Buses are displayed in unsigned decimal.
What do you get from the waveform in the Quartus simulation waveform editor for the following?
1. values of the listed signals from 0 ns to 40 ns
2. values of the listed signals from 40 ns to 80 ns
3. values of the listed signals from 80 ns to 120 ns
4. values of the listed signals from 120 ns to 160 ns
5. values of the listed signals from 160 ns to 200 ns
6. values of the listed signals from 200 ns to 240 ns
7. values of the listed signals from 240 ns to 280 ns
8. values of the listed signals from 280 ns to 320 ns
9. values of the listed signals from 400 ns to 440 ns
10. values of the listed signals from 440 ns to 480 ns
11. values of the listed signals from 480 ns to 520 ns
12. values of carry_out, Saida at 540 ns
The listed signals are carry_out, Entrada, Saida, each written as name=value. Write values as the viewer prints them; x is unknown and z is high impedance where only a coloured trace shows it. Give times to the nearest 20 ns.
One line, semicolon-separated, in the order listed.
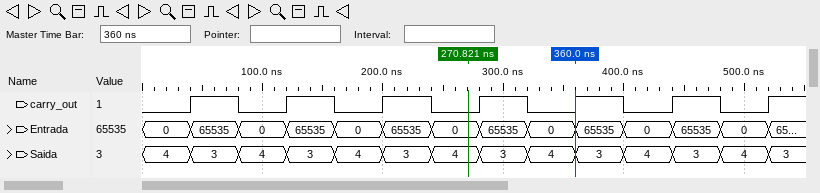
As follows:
carry_out=0, Entrada=0, Saida=4; carry_out=1, Entrada=65535, Saida=3; carry_out=0, Entrada=0, Saida=4; carry_out=1, Entrada=65535, Saida=3; carry_out=0, Entrada=0, Saida=4; carry_out=1, Entrada=65535, Saida=3; carry_out=0, Entrada=0, Saida=4; carry_out=1, Entrada=65535, Saida=3; carry_out=0, Entrada=0, Saida=4; carry_out=1, Entrada=65535, Saida=3; carry_out=0, Entrada=0, Saida=4; carry_out=1, Saida=3
